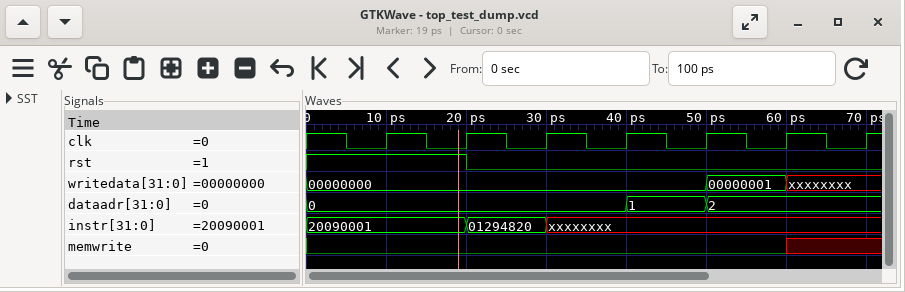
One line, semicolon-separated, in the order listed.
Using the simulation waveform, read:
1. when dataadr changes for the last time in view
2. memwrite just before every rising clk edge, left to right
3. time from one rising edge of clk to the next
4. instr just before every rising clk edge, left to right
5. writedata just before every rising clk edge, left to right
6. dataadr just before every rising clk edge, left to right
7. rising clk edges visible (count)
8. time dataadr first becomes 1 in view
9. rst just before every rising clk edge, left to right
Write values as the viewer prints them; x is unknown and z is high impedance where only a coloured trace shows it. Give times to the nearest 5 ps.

50 ps; 0 0 0 0 0 0 x; 10 ps; 20090001, 20090001, 01294820, xxxxxxxx, xxxxxxxx, xxxxxxxx, xxxxxxxx; 00000000, 00000000, 00000000, 00000000, 00000000, 00000001, xxxxxxxx; 0, 0, 0, 0, 1, 2, 2; 7; 40 ps; 1 1 0 0 0 0 0
